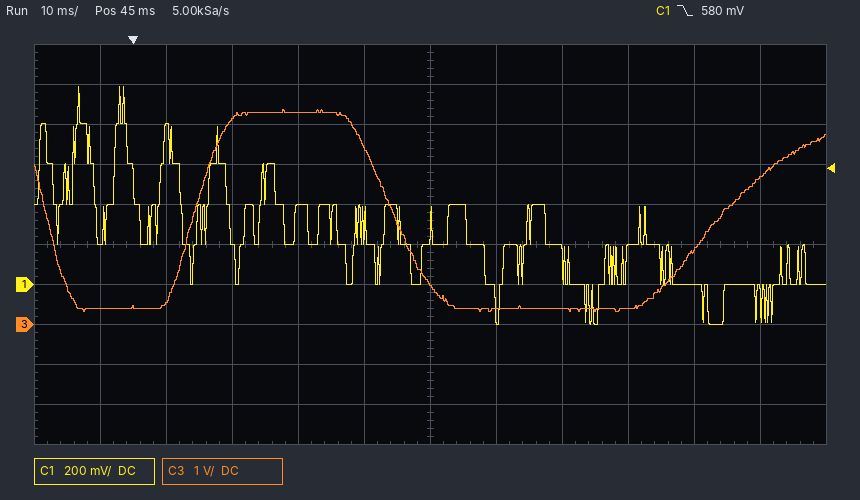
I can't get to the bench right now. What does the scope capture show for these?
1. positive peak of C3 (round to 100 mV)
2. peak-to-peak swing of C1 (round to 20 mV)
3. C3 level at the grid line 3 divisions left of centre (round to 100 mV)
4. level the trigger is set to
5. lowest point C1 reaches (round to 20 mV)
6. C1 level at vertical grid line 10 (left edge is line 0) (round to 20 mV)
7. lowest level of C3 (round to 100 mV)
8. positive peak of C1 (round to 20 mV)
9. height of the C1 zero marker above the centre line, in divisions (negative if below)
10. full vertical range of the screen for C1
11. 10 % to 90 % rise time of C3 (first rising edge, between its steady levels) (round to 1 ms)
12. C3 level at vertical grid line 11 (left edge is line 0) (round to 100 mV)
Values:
5.4 V
1.20 V
5.1 V
580 mV
-200 mV
0 mV
300 mV
1.00 V
-1.0 div
2 V
8 ms
3.7 V
